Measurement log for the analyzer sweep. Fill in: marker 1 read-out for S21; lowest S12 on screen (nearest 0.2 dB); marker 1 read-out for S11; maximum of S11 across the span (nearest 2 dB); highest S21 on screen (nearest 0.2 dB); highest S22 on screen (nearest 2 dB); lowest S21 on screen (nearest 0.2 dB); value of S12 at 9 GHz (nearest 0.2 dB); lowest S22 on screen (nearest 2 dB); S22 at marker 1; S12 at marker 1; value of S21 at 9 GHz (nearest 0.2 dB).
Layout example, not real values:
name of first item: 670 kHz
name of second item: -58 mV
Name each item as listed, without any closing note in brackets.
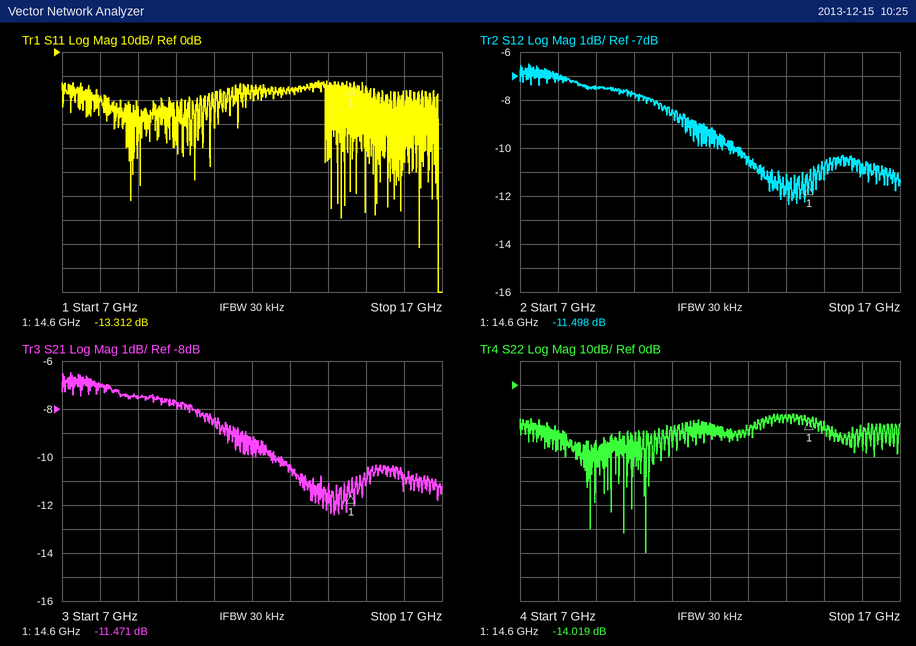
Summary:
marker 1 read-out for S21: -11.471 dB
lowest S12 on screen: -12.4 dB
marker 1 read-out for S11: -13.312 dB
maximum of S11 across the span: -12 dB
highest S21 on screen: -6.4 dB
highest S22 on screen: -12 dB
lowest S21 on screen: -12.4 dB
value of S12 at 9 GHz: -7.6 dB
lowest S22 on screen: -70 dB
S22 at marker 1: -14.019 dB
S12 at marker 1: -11.498 dB
value of S21 at 9 GHz: -7.6 dB
